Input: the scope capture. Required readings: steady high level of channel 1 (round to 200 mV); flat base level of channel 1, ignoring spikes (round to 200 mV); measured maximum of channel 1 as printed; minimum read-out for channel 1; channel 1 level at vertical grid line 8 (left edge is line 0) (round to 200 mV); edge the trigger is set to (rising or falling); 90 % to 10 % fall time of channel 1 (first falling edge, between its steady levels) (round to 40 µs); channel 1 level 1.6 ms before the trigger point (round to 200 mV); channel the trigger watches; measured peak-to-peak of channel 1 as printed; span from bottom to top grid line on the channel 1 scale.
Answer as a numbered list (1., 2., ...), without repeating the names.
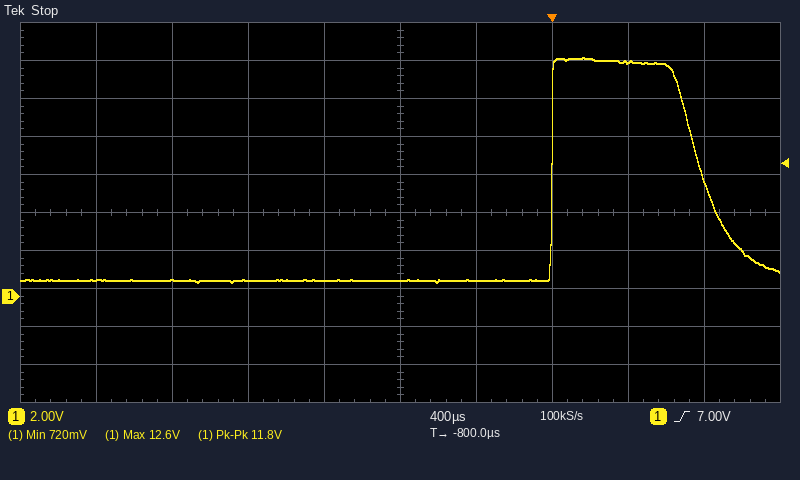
1. 12.4 V
2. 800 mV
3. 12.6 V
4. 720 mV
5. 12.4 V
6. rising
7. 400 µs
8. 800 mV
9. channel 1
10. 11.8 V
11. 20 V
